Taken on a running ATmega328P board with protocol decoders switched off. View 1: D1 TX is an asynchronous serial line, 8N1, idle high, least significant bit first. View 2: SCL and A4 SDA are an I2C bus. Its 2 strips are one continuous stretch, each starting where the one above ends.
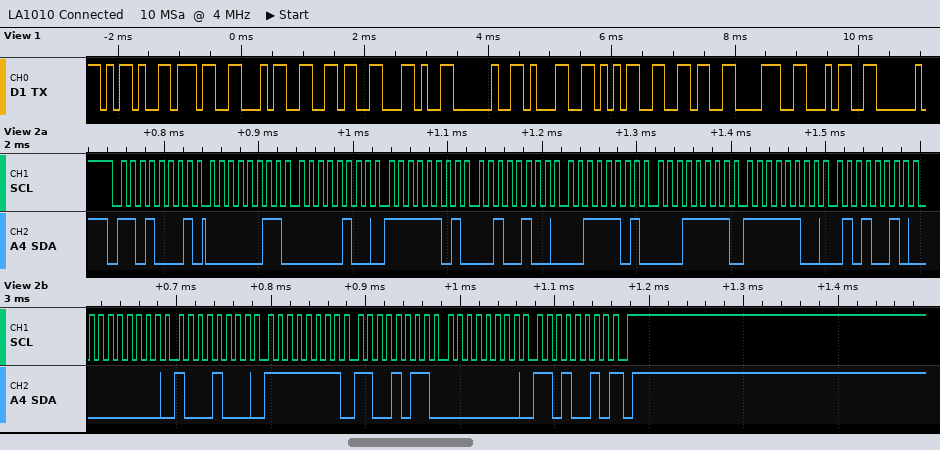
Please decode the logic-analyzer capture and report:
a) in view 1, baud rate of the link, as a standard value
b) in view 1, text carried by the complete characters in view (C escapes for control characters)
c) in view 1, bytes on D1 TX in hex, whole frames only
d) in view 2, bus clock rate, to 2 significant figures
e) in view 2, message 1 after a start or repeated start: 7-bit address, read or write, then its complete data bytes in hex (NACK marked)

9600 baud
"-746, 15684"
2D 37 34 36 2C 20 31 35 36 38 34
100 kHz
0x68 read: 03 04 FD 24 3D 1F FC 52 00 88 FF CB 00 D2 NACK
